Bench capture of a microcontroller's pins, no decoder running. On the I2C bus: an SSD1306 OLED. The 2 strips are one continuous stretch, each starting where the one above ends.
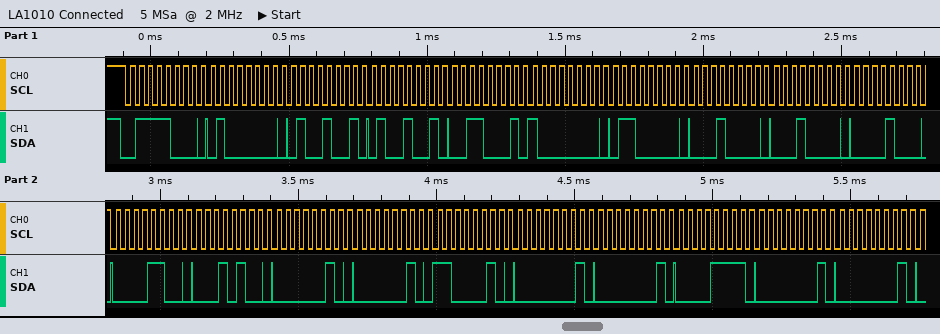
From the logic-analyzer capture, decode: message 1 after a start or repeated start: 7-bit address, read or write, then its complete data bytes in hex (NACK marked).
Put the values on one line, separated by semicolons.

0x3C write: 40 49 49 31 80 60 10 10 08 0C 14 02 02 C2 01 01 0F 01 01
